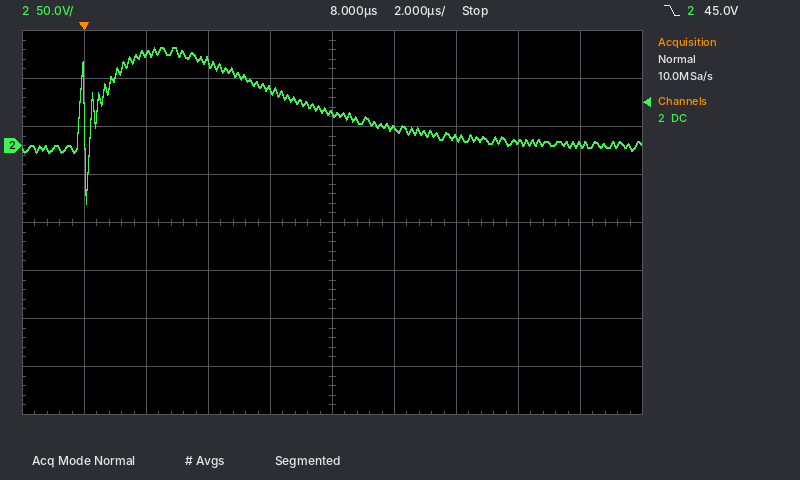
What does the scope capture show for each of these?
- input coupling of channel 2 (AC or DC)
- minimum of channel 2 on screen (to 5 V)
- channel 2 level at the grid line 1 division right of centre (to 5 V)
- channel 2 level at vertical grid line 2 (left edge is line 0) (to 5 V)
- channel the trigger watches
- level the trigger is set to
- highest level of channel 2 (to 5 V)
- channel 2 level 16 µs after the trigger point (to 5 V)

DC
-60 V
20 V
95 V
channel 2
45.0 V
100 V
0 V
